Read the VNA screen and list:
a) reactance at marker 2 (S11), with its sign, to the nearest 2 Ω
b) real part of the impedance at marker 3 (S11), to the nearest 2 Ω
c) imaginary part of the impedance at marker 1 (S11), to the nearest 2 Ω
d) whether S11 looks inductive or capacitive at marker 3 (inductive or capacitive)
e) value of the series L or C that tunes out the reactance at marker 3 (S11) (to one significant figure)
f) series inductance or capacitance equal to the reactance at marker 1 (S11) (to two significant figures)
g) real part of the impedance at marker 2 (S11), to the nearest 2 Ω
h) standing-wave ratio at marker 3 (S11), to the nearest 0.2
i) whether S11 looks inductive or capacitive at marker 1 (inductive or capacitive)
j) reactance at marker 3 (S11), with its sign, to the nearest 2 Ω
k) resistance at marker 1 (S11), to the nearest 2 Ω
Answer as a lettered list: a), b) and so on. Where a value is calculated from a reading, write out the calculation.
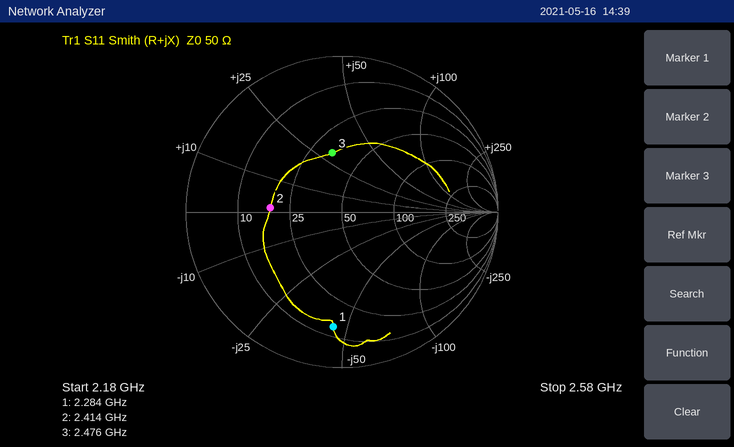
a) +2 Ω
b) 34 Ω
c) -44 Ω
d) inductive
e) C = 1/(2π × 2.476 GHz × 30 Ω) ≈ 2 pF
f) C = 1/(2π × 2.284 GHz × 44 Ω) ≈ 1.6 pF
g) 18 Ω
h) 2.2
i) capacitive
j) +30 Ω
k) 14 Ω
